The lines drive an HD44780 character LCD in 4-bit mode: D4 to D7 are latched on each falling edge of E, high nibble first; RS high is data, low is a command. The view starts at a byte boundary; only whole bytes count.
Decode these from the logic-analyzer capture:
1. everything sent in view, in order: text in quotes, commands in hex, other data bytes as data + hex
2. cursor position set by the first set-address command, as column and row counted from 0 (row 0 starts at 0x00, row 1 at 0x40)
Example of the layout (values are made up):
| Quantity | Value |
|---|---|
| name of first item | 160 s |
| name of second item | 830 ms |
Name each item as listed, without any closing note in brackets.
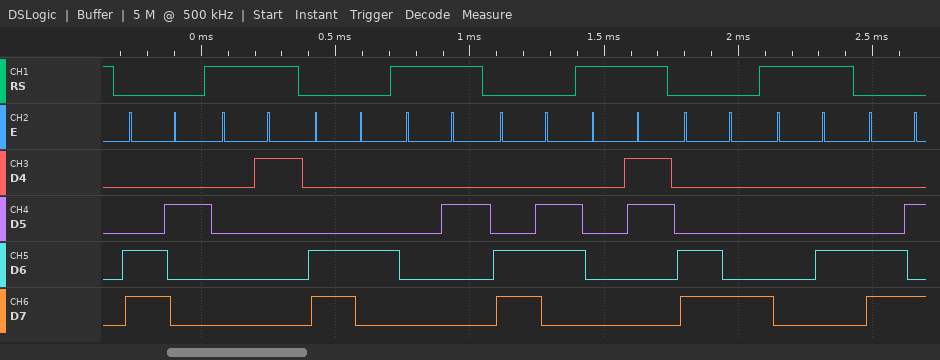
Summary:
| Quantity | Value |
|---|---|
| everything sent in view, in order: text in quotes, commands in hex, other data bytes as data + hex | 0xC2 data 01 0xC4 data 02 0xC6 data 03 0xC8 data 04 0xCA |
| cursor position set by the first set-address command, as column and row counted from 0 | column 2, row 1 |
